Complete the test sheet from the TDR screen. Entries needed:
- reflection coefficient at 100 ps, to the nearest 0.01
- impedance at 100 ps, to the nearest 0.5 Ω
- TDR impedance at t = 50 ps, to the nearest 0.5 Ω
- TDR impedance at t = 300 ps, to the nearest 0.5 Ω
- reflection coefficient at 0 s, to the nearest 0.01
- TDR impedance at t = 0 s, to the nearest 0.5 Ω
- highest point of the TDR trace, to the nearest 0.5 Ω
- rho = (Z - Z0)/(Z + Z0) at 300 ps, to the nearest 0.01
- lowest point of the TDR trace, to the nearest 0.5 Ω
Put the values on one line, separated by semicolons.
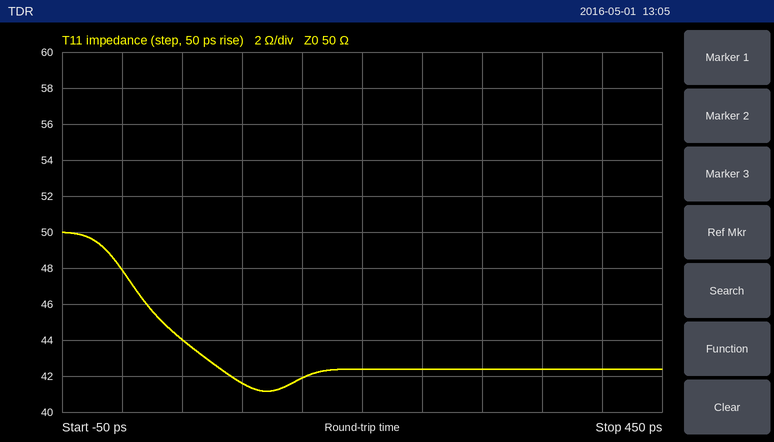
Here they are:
-0.09; 41.5 Ω; 44.0 Ω; 42.5 Ω; -0.02; 48.0 Ω; 50.0 Ω; -0.08; 41.0 Ω
